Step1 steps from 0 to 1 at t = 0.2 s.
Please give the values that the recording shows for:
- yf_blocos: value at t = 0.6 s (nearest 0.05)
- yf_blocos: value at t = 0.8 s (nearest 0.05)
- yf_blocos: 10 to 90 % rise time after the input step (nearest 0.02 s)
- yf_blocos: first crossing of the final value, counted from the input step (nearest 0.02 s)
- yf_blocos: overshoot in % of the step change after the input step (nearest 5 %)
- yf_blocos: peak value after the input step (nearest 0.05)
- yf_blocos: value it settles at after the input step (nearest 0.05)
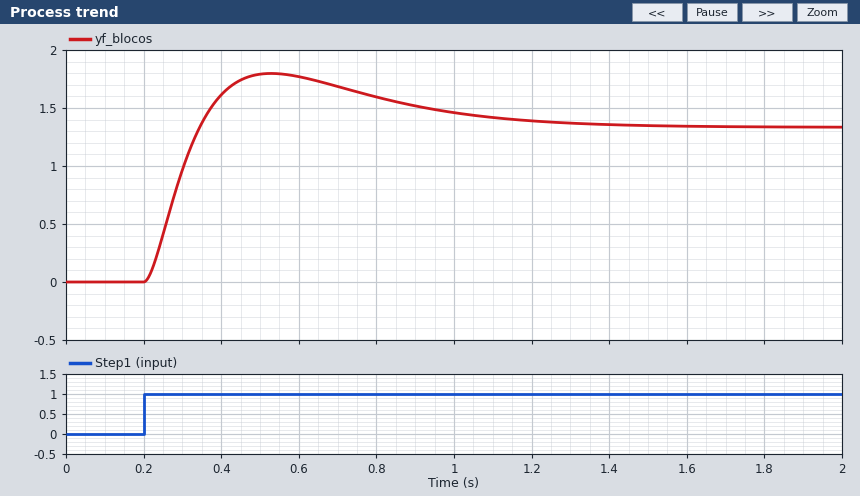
1.75
1.60
0.10 s
0.14 s
35 %
1.80
1.35
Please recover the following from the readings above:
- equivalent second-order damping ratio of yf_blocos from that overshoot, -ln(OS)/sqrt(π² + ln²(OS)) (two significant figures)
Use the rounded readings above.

0.32
